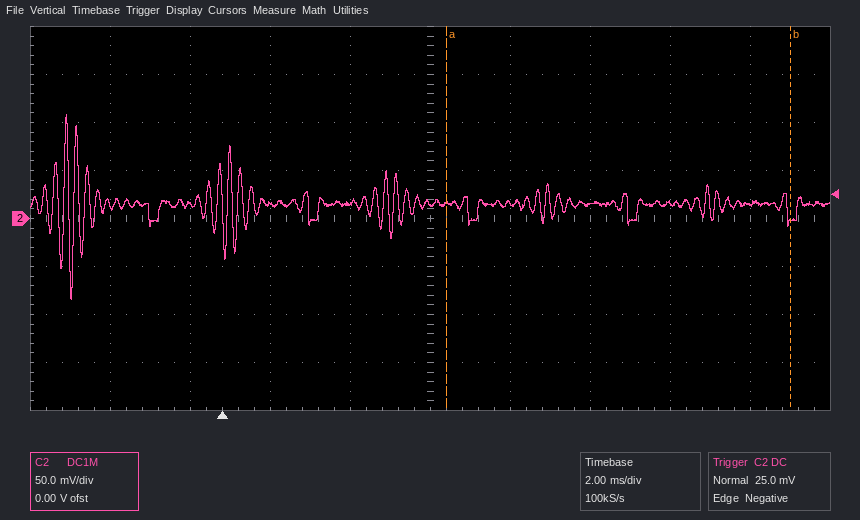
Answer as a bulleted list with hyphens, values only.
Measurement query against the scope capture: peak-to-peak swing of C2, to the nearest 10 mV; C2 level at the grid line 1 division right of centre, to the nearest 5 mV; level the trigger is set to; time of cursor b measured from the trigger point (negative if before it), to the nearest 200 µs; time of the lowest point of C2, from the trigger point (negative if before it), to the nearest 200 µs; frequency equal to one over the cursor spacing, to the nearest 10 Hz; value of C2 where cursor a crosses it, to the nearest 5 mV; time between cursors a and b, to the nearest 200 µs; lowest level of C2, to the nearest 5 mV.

- 190 mV
- 15 mV
- 25.0 mV
- +14.2 ms
- -3.8 ms
- 120 Hz
- 15 mV
- 8.6 ms
- -85 mV
